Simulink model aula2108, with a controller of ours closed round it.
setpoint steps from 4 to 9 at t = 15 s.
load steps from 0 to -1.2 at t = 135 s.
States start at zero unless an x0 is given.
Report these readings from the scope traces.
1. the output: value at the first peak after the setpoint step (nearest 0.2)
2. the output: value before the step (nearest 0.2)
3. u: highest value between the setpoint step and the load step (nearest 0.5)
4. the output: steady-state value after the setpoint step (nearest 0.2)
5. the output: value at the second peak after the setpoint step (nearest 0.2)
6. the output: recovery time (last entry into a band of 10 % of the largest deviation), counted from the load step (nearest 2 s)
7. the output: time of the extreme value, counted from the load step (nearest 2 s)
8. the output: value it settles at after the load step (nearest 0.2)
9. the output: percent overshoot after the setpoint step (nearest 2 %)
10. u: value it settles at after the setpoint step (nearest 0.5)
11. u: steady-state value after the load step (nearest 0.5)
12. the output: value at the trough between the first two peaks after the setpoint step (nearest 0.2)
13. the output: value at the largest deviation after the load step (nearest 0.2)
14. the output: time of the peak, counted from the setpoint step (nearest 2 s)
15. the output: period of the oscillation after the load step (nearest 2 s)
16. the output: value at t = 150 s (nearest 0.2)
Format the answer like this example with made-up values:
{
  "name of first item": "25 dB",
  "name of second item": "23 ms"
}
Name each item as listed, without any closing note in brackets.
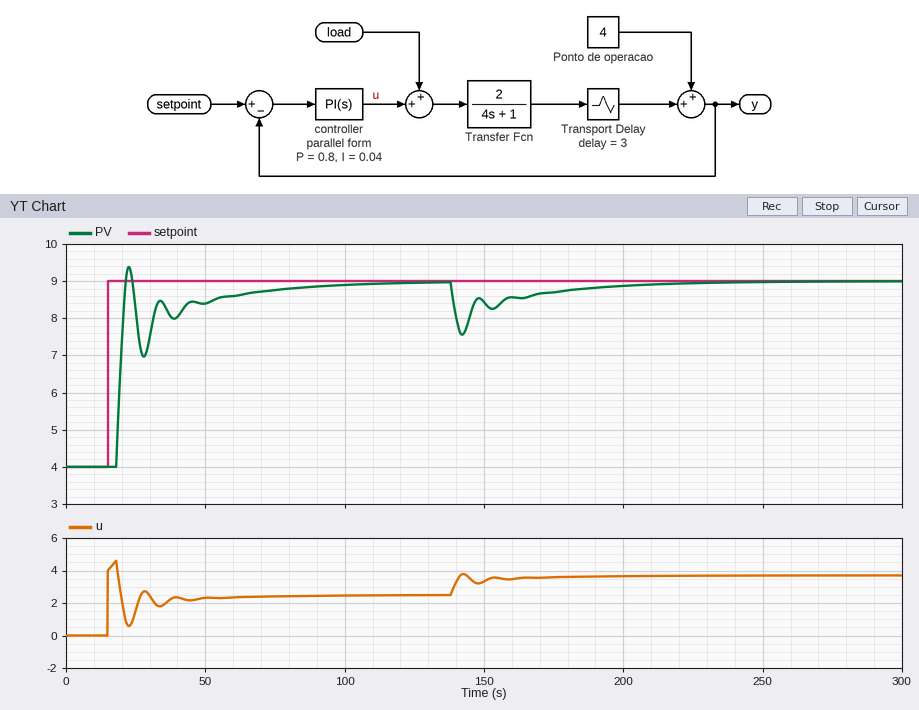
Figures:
{
  "the output: value at the first peak after the setpoint step": "9.4",
  "the output: value before the step": "4.0",
  "u: highest value between the setpoint step and the load step": "4.5",
  "the output: steady-state value after the setpoint step": "9.0",
  "the output: value at the second peak after the setpoint step": "8.4",
  "the output: recovery time (last entry into a band of 10 % of the largest deviation), counted from the load step": "62 s",
  "the output: time of the extreme value, counted from the load step": "8 s",
  "the output: value it settles at after the load step": "9.0",
  "the output: percent overshoot after the setpoint step": "8 %",
  "u: value it settles at after the setpoint step": "2.5",
  "u: steady-state value after the load step": "3.5",
  "the output: value at the trough between the first two peaks after the setpoint step": "7.0",
  "the output: value at the largest deviation after the load step": "7.6",
  "the output: time of the peak, counted from the setpoint step": "8 s",
  "the output: period of the oscillation after the load step": "10 s",
  "the output: value at t = 150 s": "8.4"
}
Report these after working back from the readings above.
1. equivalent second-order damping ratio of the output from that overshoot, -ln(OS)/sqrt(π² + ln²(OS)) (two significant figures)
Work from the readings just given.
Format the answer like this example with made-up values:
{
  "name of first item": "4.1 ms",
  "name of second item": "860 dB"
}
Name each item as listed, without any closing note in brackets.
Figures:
{
  "equivalent second-order damping ratio of the output from that overshoot, -ln(OS)/sqrt(π² + ln²(OS))": "0.63"
}
